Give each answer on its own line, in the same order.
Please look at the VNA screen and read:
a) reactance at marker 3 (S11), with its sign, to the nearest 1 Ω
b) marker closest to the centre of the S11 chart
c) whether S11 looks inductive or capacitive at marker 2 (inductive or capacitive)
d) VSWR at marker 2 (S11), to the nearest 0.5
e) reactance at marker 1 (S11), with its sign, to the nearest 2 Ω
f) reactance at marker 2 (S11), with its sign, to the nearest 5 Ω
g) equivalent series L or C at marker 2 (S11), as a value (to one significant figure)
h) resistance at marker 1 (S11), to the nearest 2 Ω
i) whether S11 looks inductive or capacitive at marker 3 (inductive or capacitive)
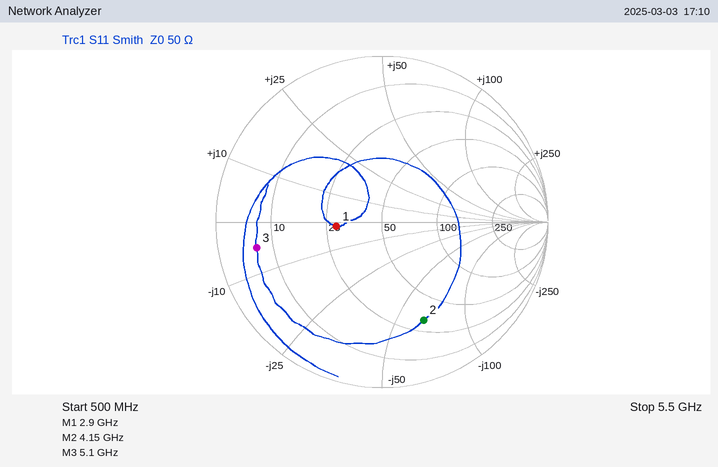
-5 Ω
marker 1
capacitive
4.5
-2 Ω
-65 Ω
600 fF
28 Ω
capacitive
